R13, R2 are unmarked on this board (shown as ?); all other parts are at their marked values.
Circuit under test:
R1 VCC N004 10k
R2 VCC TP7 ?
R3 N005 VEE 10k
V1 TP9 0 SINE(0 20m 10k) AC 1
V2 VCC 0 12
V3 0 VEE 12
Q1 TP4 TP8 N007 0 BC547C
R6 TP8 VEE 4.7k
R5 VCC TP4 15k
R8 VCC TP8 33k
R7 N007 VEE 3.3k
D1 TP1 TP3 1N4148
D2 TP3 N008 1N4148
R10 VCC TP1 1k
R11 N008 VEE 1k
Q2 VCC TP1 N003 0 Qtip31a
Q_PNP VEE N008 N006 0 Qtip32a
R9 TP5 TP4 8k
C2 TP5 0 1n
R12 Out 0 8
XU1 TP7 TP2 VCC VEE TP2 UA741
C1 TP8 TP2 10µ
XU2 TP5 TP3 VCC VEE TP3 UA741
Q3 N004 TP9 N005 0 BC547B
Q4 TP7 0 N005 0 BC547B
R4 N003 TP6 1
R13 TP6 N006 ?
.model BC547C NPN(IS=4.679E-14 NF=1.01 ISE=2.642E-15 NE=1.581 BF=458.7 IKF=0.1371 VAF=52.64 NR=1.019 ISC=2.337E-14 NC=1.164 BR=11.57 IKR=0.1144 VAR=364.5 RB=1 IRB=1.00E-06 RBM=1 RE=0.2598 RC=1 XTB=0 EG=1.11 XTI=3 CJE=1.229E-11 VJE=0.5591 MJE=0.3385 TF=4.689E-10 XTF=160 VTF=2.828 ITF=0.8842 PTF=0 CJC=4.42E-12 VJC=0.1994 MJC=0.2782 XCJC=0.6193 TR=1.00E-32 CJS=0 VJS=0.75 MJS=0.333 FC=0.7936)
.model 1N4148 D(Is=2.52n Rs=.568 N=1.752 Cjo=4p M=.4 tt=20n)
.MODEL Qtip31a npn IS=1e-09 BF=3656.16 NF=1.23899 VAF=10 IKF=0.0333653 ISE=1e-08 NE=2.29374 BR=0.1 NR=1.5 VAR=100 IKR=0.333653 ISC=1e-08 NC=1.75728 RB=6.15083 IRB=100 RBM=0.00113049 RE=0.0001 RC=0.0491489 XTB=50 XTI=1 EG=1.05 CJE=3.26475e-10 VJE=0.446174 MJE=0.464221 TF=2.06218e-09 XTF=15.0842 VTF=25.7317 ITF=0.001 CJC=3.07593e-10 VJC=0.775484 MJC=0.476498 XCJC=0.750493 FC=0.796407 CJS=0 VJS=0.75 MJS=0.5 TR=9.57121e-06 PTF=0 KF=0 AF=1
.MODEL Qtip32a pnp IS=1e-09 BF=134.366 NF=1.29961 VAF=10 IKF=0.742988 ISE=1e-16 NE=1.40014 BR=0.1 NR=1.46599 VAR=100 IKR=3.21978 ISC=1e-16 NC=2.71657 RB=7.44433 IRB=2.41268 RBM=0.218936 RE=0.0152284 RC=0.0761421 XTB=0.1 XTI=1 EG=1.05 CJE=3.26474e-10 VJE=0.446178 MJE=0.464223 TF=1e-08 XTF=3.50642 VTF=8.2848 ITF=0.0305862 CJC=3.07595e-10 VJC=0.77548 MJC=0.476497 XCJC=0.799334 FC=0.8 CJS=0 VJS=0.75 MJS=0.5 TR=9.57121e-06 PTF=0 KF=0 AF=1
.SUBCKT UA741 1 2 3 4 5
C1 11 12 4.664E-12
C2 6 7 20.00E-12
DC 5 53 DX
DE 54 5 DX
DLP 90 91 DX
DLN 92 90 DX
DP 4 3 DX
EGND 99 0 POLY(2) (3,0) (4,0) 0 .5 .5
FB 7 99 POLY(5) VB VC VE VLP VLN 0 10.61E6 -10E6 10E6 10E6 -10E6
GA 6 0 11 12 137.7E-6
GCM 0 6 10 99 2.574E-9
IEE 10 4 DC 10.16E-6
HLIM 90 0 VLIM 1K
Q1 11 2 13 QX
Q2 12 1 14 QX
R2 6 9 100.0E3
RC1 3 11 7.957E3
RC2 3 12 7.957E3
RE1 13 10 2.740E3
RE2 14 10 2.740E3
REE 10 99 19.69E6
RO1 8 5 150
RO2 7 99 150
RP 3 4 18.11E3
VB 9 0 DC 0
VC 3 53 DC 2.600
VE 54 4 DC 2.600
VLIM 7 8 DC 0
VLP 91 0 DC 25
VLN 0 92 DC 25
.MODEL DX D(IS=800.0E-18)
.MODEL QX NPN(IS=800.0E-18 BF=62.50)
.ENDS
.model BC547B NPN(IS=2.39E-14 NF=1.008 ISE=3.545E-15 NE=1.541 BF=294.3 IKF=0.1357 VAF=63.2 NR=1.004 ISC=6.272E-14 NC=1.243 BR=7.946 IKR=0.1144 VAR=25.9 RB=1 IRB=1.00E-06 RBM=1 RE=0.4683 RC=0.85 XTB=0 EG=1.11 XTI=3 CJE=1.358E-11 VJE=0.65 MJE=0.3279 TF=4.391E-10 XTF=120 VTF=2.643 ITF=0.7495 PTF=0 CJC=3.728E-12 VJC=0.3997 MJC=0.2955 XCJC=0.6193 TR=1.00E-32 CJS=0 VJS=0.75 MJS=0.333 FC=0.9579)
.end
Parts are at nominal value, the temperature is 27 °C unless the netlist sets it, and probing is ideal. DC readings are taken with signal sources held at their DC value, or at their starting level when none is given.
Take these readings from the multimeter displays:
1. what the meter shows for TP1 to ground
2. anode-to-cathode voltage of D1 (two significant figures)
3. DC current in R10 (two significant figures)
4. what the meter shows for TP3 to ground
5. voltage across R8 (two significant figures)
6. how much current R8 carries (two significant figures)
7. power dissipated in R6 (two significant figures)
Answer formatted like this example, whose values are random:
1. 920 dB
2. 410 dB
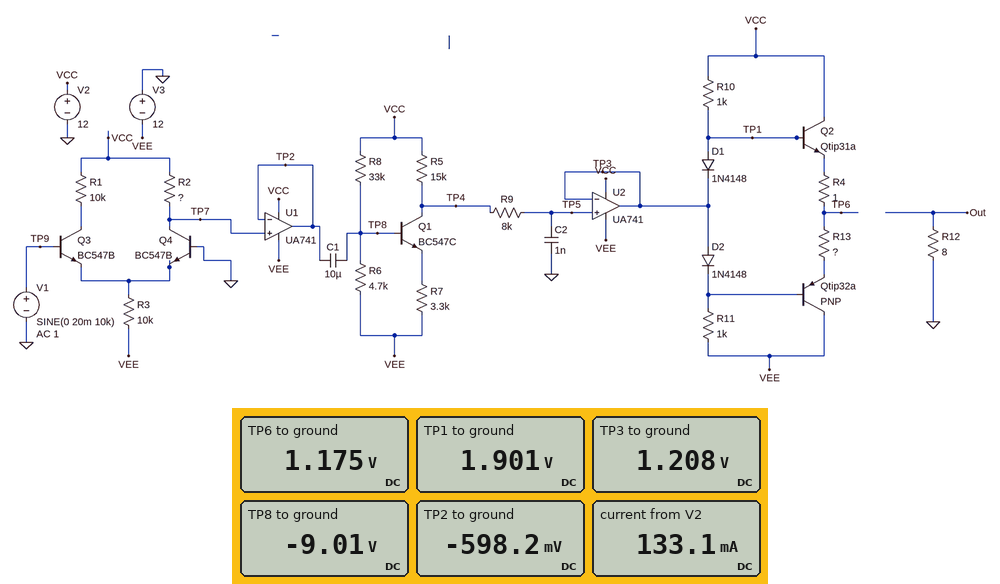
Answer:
1. 1.901 V
2. 690 mV
3. 10 mA
4. 1.208 V
5. 21 V
6. 640 µA
7. 1.9 mW
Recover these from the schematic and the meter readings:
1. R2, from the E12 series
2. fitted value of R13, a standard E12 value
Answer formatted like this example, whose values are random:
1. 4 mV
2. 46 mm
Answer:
1. 33 kΩ
2. 0.56 Ω
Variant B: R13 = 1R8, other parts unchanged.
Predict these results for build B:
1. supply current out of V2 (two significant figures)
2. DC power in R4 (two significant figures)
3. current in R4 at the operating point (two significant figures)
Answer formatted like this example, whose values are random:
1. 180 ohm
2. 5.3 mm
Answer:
1. 94 mA
2. 6.3 mW
3. 79 mA
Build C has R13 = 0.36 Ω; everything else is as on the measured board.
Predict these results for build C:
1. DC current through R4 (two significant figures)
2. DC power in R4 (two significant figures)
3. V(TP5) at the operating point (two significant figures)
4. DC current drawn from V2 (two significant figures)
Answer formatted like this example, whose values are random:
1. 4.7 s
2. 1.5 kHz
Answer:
1. 130 mA
2. 17 mW
3. 1.2 V
4. 140 mA
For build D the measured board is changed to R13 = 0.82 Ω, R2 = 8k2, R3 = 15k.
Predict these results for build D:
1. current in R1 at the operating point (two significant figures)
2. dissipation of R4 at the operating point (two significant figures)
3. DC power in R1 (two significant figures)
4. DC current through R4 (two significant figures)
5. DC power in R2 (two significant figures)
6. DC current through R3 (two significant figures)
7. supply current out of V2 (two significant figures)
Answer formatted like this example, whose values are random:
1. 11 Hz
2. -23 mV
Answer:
1. 380 µA
2. 11 mW
3. 1.4 mW
4. 110 mA
5. 1.2 mW
6. 760 µA
7. 120 mA
